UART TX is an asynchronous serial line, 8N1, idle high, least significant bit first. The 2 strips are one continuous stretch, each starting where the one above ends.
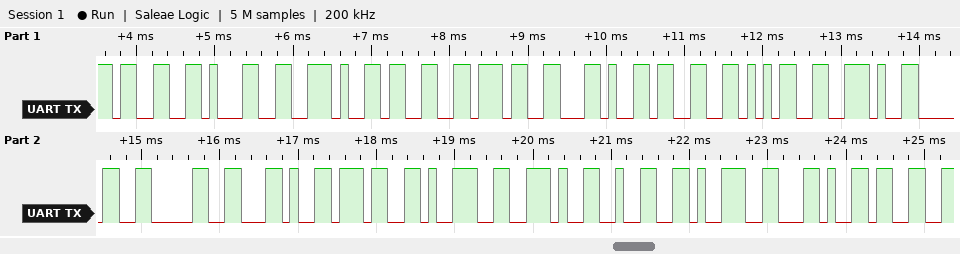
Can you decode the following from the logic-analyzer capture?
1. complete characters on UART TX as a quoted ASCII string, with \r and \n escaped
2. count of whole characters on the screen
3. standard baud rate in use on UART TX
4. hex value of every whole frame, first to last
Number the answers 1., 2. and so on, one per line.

1. "31.37,35.00,79.29,3"
2. 19
3. 9600 baud
4. 33 31 2E 33 37 2C 33 35 2E 30 30 2C 37 39 2E 32 39 2C 33
